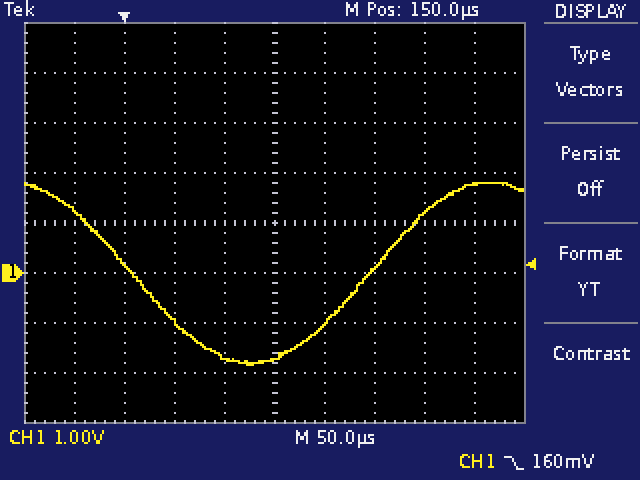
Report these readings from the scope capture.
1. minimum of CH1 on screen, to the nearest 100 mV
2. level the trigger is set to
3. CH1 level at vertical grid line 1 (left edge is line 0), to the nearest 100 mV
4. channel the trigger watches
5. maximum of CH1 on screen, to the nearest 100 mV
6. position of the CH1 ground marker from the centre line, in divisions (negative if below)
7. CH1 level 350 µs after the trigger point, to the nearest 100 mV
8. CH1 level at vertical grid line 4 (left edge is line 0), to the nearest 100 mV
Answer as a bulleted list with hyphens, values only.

- -1.8 V
- 160 mV
- 1.2 V
- CH1
- 1.8 V
- -1.0 div
- 1.8 V
- -1.7 V
